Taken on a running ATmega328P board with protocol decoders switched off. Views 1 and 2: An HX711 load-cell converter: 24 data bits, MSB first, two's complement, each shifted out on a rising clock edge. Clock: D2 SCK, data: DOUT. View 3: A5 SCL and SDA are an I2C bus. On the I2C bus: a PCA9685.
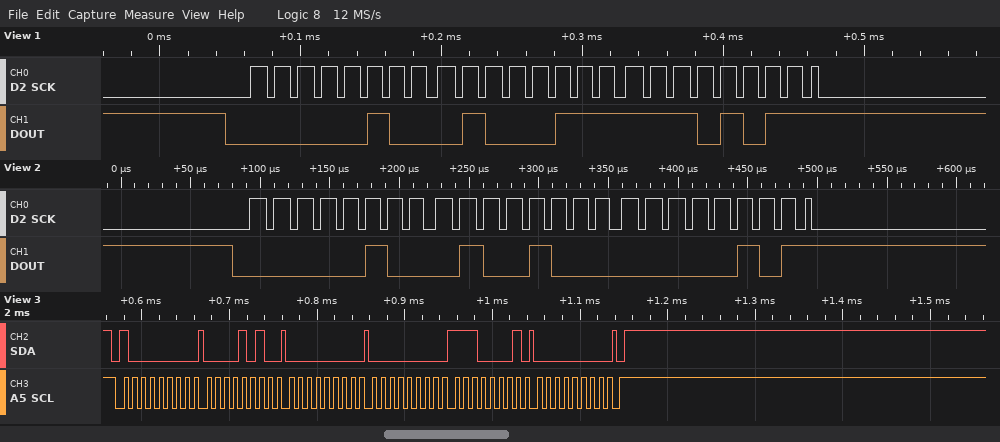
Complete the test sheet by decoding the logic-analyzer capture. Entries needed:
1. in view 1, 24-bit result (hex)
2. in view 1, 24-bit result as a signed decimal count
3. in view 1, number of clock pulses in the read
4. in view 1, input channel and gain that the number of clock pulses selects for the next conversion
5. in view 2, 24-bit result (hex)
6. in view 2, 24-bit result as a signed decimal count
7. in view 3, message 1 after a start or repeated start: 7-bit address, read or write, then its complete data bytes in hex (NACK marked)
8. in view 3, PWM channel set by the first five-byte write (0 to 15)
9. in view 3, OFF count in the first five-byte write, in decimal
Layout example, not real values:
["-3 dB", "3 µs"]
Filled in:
["0x0447EB", "280555", "25", "channel A, gain 128", "0x044805", "280581", "0x40 write: 0A 00 00 E1 00", "1", "225"]
